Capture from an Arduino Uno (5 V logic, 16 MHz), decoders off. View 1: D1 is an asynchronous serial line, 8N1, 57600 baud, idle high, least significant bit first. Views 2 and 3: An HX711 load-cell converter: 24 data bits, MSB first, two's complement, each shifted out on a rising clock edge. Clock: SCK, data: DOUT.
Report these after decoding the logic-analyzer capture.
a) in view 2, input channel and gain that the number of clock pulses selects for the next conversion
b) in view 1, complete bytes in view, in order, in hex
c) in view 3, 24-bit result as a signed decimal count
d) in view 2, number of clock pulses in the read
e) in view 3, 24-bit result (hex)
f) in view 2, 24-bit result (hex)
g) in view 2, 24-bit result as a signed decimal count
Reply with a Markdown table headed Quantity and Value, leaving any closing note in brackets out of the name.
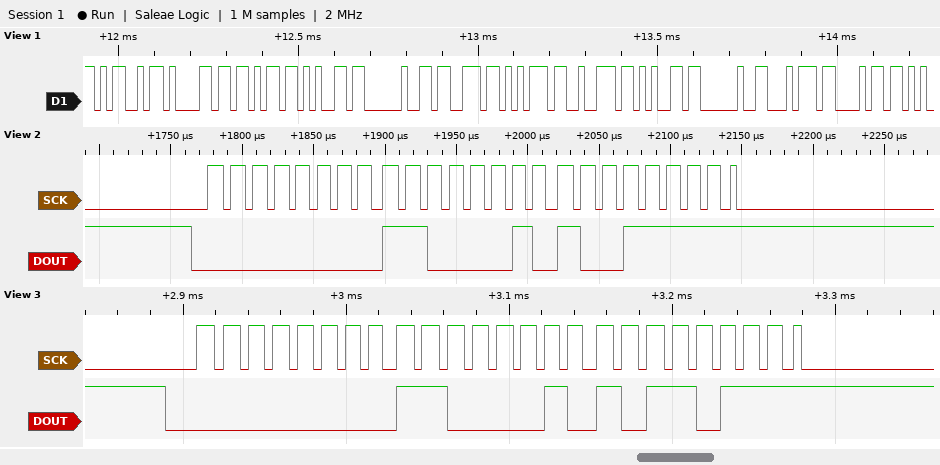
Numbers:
| Quantity | Value |
|---|---|
| in view 2, input channel and gain that the number of clock pulses selects for the next conversion | channel A, gain 128 |
| in view 1, complete bytes in view, in order, in hex | 4D 61 6B 65 20 73 75 72 65 20 74 68 |
| in view 3, 24-bit result as a signed decimal count | 49847 |
| in view 2, number of clock pulses in the read | 25 |
| in view 3, 24-bit result | 0x00C2B7 |
| in view 2, 24-bit result | 0x00C29F |
| in view 2, 24-bit result as a signed decimal count | 49823 |
